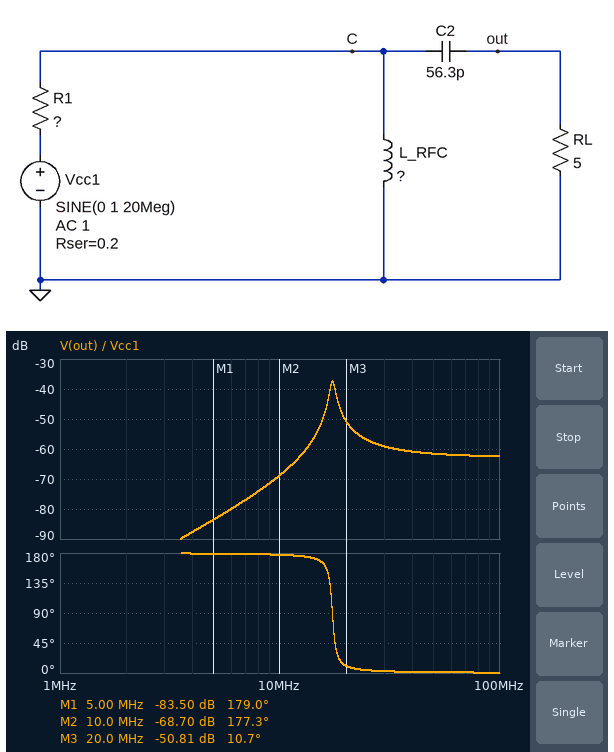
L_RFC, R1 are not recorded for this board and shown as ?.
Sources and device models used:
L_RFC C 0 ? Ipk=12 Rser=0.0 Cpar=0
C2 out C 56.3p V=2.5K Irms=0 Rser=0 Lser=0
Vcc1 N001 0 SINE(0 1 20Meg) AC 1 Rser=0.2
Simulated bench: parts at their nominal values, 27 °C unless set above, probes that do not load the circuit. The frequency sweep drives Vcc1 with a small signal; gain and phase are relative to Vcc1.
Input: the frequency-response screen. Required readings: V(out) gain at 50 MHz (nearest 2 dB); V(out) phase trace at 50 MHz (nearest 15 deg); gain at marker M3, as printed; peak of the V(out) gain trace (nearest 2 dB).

-62 dB
0 deg
-50.81 dB
-38 dB
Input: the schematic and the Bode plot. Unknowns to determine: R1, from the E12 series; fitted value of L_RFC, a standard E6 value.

6.8 kΩ
1.5 µH
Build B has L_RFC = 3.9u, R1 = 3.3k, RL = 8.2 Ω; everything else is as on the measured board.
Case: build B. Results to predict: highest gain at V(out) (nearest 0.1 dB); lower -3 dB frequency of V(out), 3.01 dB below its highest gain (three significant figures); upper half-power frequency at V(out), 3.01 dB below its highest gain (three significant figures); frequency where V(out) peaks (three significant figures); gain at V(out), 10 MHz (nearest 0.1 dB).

-33.0 dB
10.2 MHz
11.4 MHz
10.8 MHz
-37.8 dB
